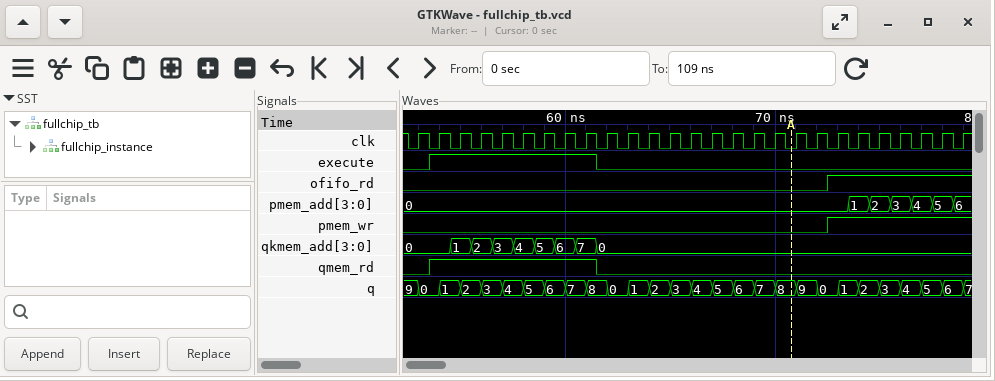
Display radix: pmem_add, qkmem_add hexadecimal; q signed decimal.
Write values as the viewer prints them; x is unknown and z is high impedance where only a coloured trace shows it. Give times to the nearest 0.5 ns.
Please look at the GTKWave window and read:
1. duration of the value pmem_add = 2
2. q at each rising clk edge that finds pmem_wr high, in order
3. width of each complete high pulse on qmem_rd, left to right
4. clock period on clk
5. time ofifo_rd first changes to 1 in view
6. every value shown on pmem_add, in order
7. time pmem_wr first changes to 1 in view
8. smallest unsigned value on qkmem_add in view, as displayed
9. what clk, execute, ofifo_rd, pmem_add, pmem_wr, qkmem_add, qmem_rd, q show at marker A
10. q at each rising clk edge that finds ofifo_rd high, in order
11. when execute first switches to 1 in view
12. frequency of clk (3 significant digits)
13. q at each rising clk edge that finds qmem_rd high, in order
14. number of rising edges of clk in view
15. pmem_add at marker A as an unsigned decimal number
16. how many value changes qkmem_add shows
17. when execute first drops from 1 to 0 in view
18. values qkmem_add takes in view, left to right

1 ns
0, 1, 2, 3, 4, 5, 6
8 ns
1 ns
72.5 ns
0, 1, 2, 3, 4, 5, 6
72.5 ns
0
clk=0, execute=0, ofifo_rd=0, pmem_add=0, pmem_wr=0, qkmem_add=0, qmem_rd=0, q=8
0, 1, 2, 3, 4, 5, 6
53.5 ns
1.00 GHz
0, 1, 2, 3, 4, 5, 6, 7
27
0
8
61.5 ns
0, 1, 2, 3, 4, 5, 6, 7, 0
